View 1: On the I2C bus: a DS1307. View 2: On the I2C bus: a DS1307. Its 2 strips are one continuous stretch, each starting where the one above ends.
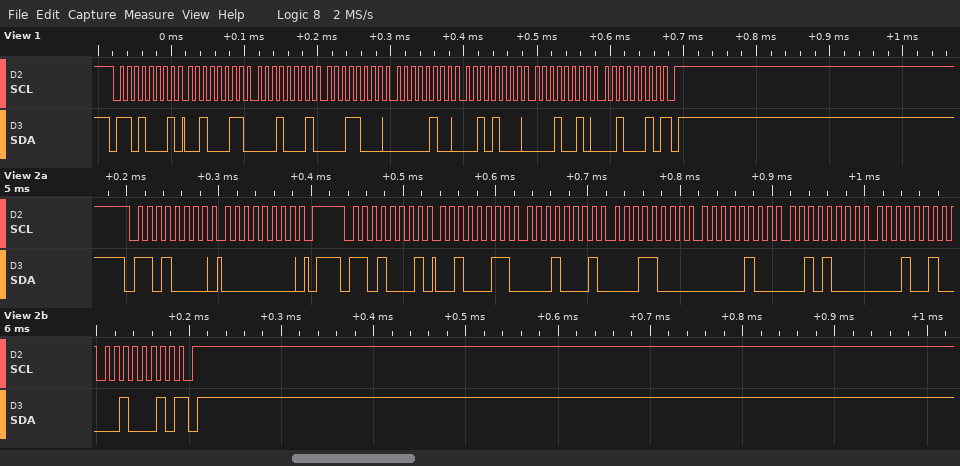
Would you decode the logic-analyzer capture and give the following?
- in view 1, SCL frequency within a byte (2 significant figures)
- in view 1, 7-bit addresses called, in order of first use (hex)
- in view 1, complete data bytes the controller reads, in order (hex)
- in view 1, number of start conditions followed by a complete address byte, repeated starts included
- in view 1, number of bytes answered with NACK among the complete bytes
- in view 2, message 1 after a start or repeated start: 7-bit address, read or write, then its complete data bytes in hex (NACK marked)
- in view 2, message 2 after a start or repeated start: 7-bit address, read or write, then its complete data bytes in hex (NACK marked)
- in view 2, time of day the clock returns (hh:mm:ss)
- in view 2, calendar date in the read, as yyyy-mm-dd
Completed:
100 kHz
0x68
23 11 18 04 28 12 22
1
1
0x68 write: 00
0x68 read: 23 11 18 04 28 12 22 NACK
18:11:23
2022-12-28
